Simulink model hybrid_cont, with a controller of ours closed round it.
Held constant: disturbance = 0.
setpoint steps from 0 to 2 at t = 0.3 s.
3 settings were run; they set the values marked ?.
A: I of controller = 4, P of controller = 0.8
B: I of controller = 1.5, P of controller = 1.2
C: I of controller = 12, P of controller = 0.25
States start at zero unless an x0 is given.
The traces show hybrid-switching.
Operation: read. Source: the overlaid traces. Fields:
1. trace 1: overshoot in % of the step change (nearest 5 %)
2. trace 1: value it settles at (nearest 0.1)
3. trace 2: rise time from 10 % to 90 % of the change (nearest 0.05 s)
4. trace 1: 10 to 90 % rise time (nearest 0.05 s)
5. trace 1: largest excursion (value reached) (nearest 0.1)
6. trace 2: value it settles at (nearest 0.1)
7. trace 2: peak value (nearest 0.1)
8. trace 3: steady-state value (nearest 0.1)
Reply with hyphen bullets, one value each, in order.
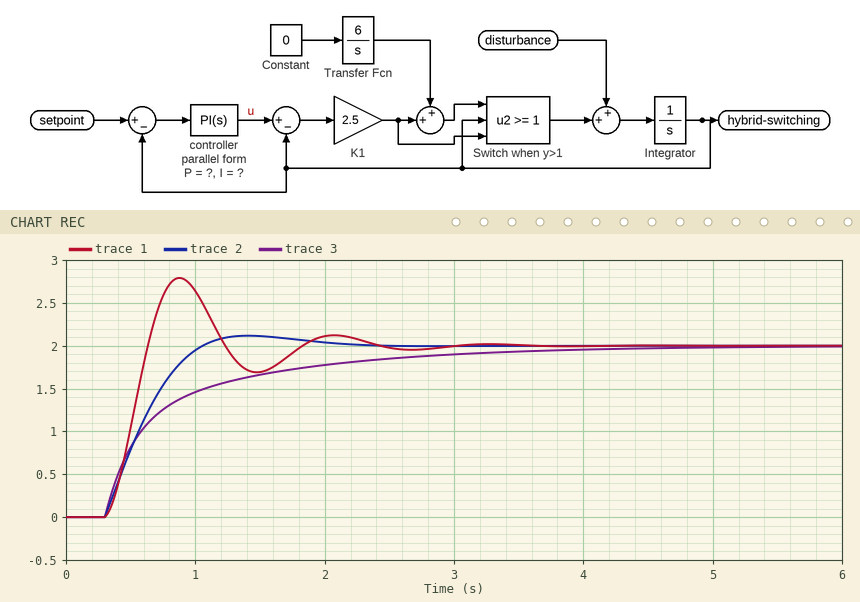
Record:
- 40 %
- 2.0
- 0.55 s
- 0.25 s
- 2.8
- 2.0
- 2.1
- 2.0
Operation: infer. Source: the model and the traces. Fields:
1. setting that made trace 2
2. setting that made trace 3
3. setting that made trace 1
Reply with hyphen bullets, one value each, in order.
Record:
- A
- B
- C
